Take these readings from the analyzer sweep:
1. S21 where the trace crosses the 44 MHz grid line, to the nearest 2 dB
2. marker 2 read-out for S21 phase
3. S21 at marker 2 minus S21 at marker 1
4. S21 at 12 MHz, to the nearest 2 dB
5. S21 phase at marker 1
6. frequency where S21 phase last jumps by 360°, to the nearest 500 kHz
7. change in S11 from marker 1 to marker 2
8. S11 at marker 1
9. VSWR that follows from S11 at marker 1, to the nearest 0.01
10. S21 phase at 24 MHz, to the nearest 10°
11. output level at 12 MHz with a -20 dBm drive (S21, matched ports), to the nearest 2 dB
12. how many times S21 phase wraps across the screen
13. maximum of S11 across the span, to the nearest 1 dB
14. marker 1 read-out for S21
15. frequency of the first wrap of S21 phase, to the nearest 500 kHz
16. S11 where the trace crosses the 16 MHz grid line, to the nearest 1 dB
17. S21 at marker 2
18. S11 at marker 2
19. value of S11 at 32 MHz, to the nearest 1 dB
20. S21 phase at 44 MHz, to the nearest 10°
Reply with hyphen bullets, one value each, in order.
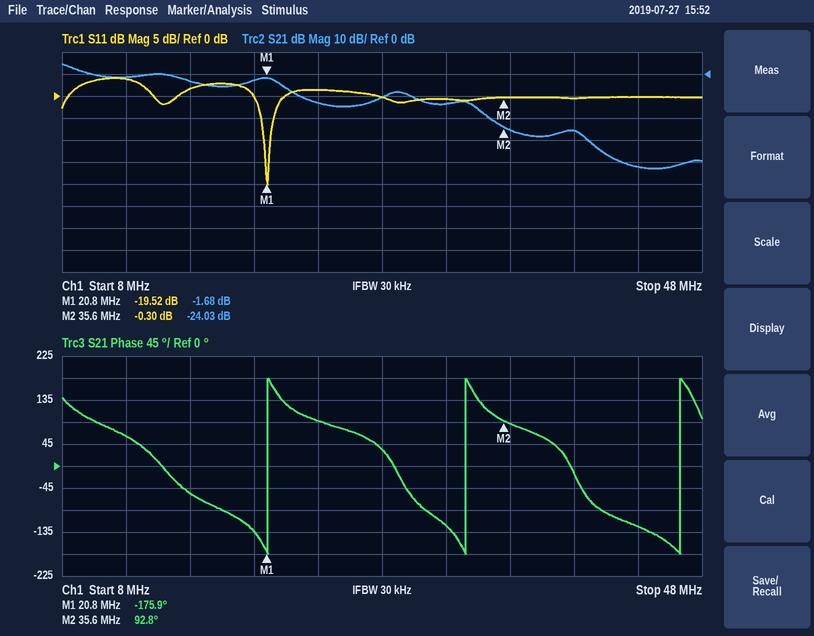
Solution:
- -42 dB
- 92.8°
- -22.35 dB
- -2 dB
- -175.9°
- 46.5 MHz
- 19.22 dB
- -19.52 dB
- 1.24
- 90°
- -22 dBm
- 3
- 4 dB
- -1.68 dB
- 21.0 MHz
- 2 dB
- -24.03 dB
- -0.30 dB
- -1 dB
- -120°
